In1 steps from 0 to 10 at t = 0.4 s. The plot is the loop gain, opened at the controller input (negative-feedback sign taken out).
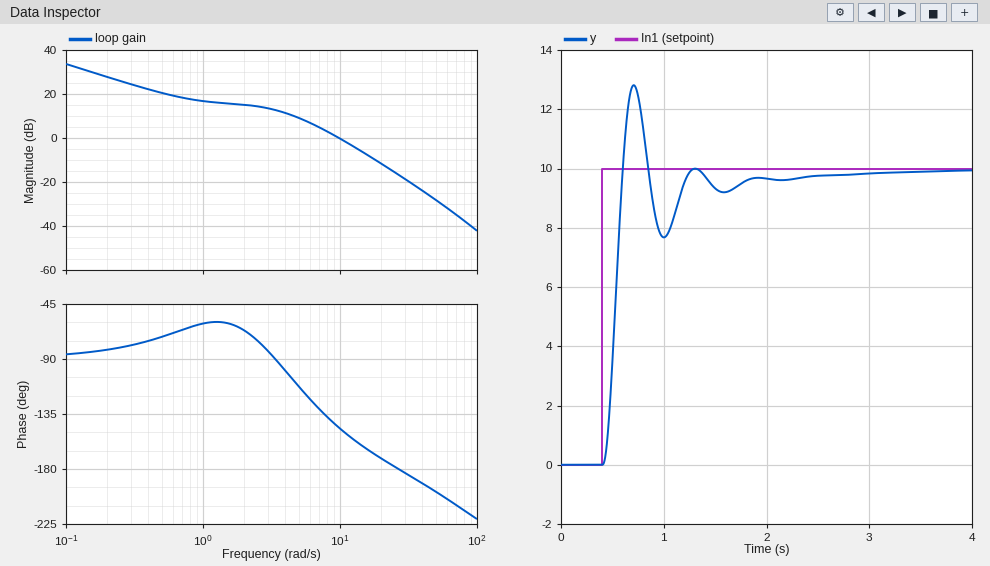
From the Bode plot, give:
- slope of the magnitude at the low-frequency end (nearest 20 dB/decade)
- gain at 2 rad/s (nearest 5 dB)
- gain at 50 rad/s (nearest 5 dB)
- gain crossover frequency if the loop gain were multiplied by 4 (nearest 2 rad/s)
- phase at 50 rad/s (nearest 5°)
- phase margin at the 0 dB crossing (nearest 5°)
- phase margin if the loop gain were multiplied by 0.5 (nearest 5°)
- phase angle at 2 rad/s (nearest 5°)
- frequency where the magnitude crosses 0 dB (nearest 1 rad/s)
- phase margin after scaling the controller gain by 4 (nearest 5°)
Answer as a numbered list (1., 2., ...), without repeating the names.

1. -20 dB/decade
2. 15 dB
3. -30 dB
4. 20 rad/s
5. -200°
6. 35°
7. 55°
8. -65°
9. 10 rad/s
10. 10°
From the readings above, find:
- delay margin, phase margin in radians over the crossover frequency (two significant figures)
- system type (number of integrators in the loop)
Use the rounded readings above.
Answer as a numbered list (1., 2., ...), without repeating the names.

1. 0.061 s
2. 1
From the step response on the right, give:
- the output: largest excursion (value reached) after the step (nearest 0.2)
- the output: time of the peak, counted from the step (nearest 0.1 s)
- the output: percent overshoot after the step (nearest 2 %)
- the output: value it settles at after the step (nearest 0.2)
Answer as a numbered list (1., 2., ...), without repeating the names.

1. 12.8
2. 0.3 s
3. 28 %
4. 10.0
